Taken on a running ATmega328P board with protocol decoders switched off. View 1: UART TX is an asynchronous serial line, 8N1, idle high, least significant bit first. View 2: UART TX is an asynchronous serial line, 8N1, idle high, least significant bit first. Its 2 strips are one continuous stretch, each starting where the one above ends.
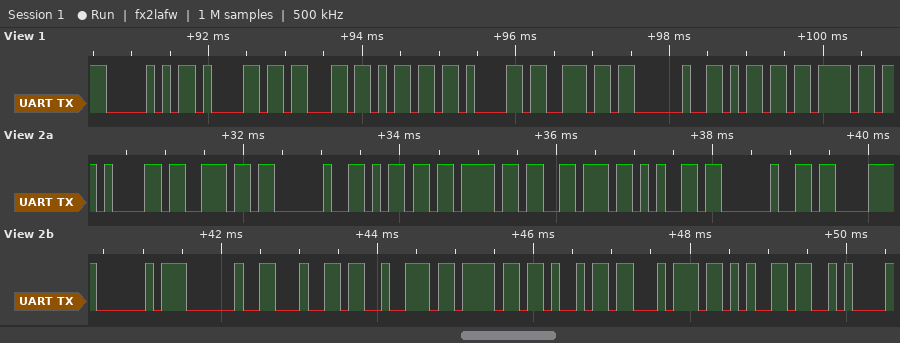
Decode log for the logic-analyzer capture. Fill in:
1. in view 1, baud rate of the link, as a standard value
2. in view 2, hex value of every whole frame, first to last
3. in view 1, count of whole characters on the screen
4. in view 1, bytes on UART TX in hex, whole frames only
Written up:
9600 baud
61 6E 20 6D 6F 76 65 20 C3 A0 20 64 72 6F 69 74 65 0A
9
0x50 0x61 0x63 0x6D 0x61 0x6E 0x20 0x6D 0x6F
